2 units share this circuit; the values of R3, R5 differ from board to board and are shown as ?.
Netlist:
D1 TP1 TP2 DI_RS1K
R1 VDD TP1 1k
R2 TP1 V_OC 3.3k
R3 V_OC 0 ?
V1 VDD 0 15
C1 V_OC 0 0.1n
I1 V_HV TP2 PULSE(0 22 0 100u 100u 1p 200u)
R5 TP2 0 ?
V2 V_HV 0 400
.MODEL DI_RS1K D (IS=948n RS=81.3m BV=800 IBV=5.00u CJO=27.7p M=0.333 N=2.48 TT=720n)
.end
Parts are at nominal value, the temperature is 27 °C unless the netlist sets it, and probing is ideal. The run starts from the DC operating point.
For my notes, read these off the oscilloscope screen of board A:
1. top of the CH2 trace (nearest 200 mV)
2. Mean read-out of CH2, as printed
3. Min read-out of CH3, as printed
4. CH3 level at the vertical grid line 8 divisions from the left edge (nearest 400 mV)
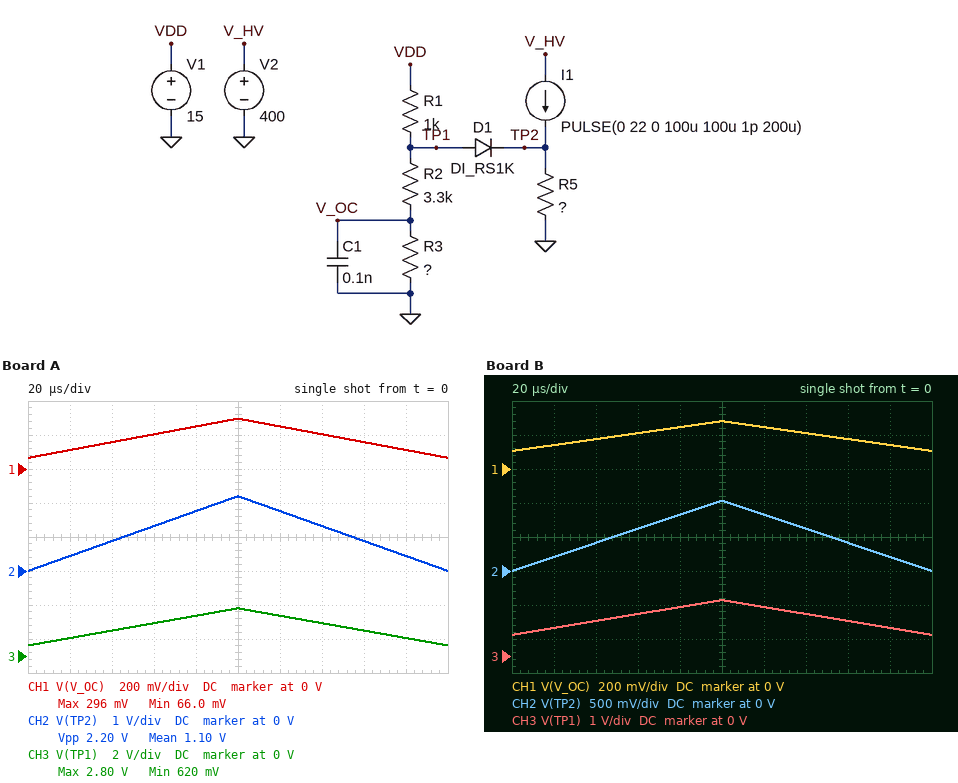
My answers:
2.2 V
1.10 V
620 mV
1.6 V
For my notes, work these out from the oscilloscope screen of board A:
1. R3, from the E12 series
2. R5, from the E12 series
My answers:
390 Ω
0.1 Ω
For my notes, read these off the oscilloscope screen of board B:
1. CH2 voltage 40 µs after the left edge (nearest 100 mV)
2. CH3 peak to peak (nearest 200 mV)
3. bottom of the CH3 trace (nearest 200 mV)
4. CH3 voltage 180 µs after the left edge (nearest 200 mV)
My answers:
400 mV
1.0 V
600 mV
800 mV
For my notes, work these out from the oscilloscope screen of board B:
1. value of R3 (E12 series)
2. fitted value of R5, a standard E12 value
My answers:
680 Ω
0.047 Ω
